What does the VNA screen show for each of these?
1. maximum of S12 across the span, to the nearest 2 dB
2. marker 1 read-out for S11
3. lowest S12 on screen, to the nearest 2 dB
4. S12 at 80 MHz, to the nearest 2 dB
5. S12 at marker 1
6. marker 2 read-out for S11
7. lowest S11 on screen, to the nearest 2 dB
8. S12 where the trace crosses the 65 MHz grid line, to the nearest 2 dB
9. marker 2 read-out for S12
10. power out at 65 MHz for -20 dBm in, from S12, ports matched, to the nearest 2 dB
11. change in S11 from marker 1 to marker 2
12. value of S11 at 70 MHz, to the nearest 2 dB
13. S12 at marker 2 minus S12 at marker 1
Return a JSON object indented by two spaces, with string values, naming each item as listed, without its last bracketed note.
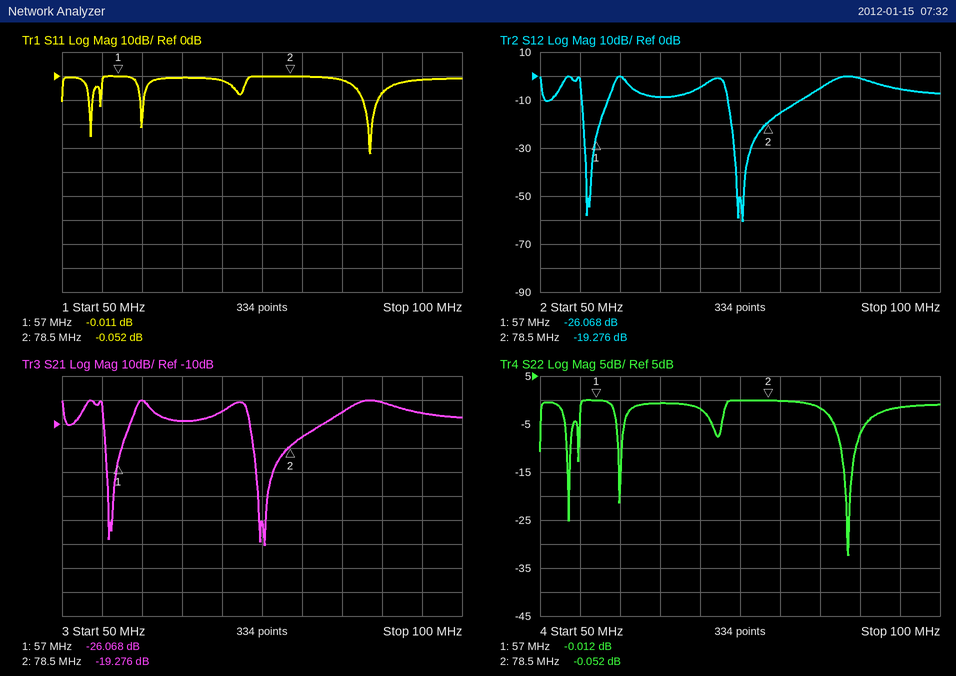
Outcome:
{
  "maximum of S12 across the span, to the nearest 2 dB": "0 dB",
  "marker 1 read-out for S11": "-0.011 dB",
  "lowest S12 on screen, to the nearest 2 dB": "-60 dB",
  "S12 at 80 MHz, to the nearest 2 dB": "-16 dB",
  "S12 at marker 1": "-26.068 dB",
  "marker 2 read-out for S11": "-0.052 dB",
  "lowest S11 on screen, to the nearest 2 dB": "-32 dB",
  "S12 where the trace crosses the 65 MHz grid line, to the nearest 2 dB": "-8 dB",
  "marker 2 read-out for S12": "-19.276 dB",
  "power out at 65 MHz for -20 dBm in, from S12, ports matched, to the nearest 2 dB": "-28 dBm",
  "change in S11 from marker 1 to marker 2": "-0.041 dB",
  "value of S11 at 70 MHz, to the nearest 2 dB": "-2 dB",
  "S12 at marker 2 minus S12 at marker 1": "6.792 dB"
}
